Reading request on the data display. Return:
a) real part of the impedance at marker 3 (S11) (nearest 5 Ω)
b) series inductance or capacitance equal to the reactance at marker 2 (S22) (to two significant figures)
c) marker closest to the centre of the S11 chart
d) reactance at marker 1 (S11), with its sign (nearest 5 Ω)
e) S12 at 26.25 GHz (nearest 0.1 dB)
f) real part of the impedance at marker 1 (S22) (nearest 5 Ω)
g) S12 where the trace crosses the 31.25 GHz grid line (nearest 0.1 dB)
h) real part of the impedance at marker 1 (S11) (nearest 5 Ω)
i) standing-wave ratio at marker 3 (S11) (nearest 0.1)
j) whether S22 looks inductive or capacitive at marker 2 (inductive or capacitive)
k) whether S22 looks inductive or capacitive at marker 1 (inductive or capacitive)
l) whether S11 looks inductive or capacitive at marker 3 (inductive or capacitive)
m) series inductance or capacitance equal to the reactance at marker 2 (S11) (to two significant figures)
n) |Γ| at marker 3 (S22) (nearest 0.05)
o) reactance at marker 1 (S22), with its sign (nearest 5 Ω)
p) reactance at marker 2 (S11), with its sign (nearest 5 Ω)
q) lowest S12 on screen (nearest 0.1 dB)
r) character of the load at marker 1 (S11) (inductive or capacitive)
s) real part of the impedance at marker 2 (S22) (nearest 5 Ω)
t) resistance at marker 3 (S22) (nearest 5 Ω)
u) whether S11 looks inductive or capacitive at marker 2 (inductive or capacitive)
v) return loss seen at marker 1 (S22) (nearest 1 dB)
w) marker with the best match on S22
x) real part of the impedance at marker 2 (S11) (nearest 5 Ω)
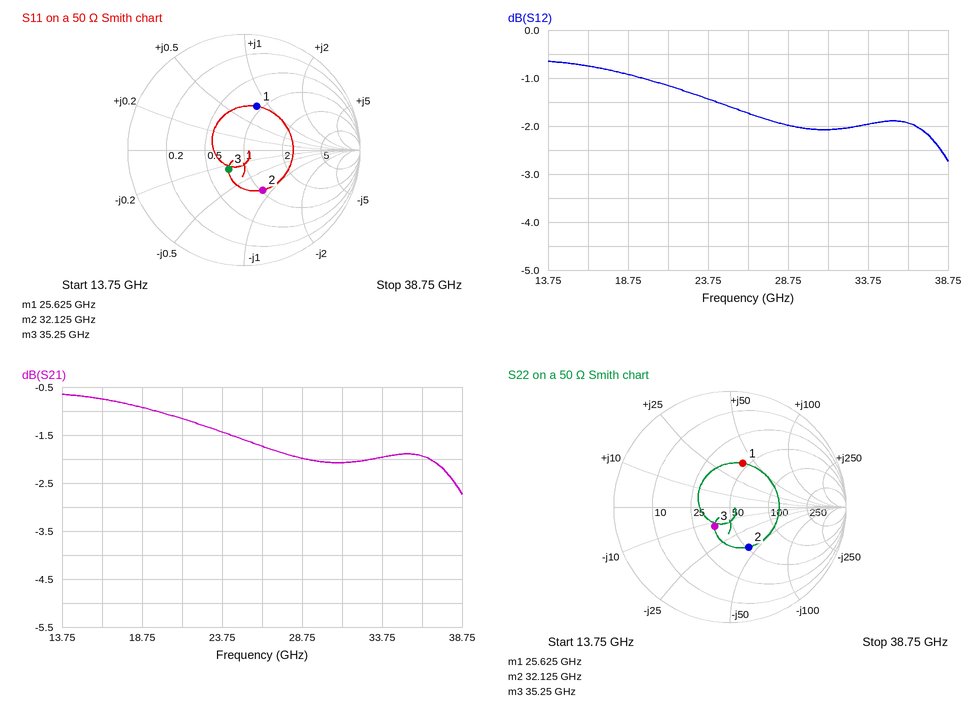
35 Ω
120 fF
marker 3
+40 Ω
-1.7 dB
45 Ω
-2.1 dB
45 Ω
1.5
capacitive
inductive
capacitive
120 fF
0.20
+40 Ω
-40 Ω
-2.7 dB
inductive
50 Ω
35 Ω
capacitive
8 dB
marker 3
50 Ω
